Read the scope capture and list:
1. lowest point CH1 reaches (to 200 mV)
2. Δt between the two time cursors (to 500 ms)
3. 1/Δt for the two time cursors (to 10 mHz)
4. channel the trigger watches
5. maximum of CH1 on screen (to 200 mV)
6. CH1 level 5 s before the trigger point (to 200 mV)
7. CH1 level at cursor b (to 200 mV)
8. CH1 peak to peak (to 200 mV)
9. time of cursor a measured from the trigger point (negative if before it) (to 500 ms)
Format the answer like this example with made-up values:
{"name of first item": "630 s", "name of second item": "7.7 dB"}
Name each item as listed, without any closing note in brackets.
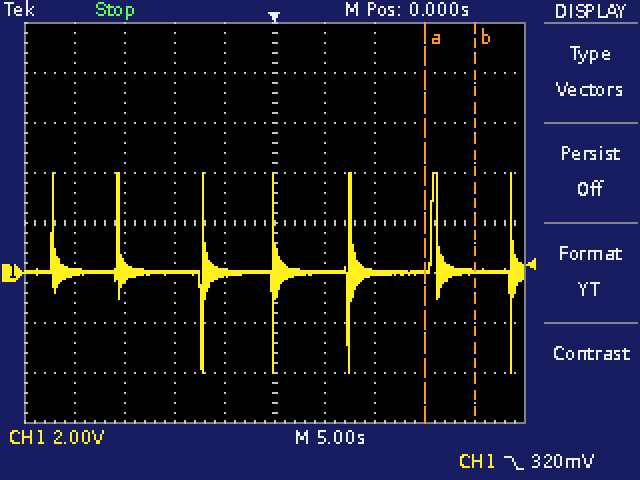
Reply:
{"lowest point CH1 reaches": "-4.0 V", "Δt between the two time cursors": "5.0 s", "1/Δt for the two time cursors": "200 mHz", "channel the trigger watches": "CH1", "maximum of CH1 on screen": "4.0 V", "CH1 level 5 s before the trigger point": "0.0 V", "CH1 level at cursor b": "0.0 V", "CH1 peak to peak": "8.0 V", "time of cursor a measured from the trigger point (negative if before it)": "+15.0 s"}
